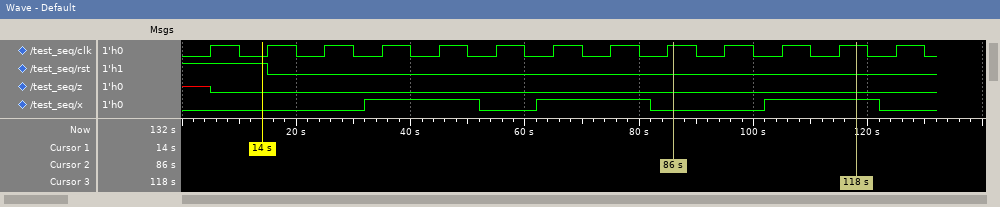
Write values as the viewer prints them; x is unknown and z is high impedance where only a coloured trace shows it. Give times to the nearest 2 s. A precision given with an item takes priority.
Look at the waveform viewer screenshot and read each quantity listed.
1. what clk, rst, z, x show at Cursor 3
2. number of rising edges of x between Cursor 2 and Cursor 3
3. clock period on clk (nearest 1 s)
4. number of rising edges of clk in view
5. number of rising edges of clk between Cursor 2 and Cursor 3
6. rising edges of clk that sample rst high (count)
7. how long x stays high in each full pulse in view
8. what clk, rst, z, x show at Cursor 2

clk=1, rst=0, z=0, x=1
1
10 s
13
3
2
20 s, 20 s, 20 s
clk=1, rst=0, z=0, x=0
